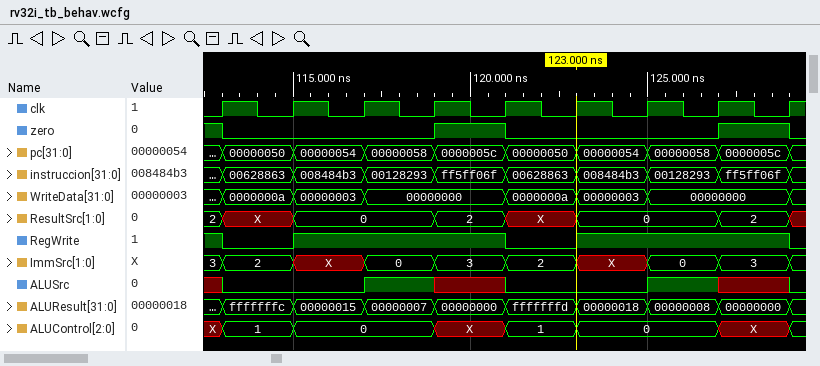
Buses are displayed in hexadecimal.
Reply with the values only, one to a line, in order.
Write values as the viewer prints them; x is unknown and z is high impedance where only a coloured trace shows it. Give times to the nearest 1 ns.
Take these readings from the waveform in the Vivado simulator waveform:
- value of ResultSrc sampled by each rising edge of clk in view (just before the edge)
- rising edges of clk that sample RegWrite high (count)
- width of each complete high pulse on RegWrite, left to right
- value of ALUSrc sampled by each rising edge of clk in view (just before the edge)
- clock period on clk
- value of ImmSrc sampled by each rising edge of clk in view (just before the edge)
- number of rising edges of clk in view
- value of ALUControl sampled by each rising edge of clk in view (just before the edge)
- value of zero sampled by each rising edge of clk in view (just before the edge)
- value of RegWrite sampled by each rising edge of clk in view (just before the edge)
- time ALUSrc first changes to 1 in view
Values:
2, X, 0, 0, 2, X, 0, 0, 2
7
6 ns, 6 ns
x 0 0 1 x 0 0 1 x
2 ns
3, 2, X, 0, 3, 2, X, 0, 3
9
X, 1, 0, 0, X, 1, 0, 0, X
1 0 0 0 1 0 0 0 1
1 0 1 1 1 0 1 1 1
117 ns
